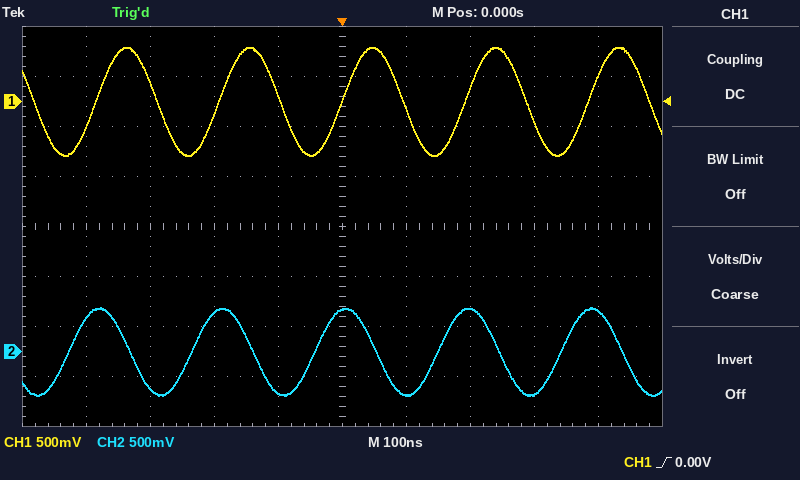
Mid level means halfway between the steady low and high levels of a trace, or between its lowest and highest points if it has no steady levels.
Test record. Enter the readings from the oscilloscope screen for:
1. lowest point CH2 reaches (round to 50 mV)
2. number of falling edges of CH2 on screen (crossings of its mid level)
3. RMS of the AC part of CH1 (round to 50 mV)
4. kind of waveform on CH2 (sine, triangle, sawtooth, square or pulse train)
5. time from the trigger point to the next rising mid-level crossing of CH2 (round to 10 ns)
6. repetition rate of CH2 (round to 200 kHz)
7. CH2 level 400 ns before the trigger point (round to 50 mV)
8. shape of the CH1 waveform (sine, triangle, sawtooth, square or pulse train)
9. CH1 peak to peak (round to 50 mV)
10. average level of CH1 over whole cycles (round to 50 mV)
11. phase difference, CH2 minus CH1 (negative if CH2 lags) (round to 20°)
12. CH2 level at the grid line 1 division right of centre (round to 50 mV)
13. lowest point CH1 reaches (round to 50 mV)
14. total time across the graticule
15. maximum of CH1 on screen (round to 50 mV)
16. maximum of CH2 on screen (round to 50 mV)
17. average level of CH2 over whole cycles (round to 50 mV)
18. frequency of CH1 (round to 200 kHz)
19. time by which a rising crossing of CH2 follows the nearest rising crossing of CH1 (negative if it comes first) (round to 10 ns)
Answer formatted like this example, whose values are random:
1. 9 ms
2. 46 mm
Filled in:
1. -450 mV
2. 5
3. 400 mV
4. sine
5. 150 ns
6. 5.2 MHz
7. 350 mV
8. sine
9. 1.10 V
10. 0 mV
11. +80°
12. -450 mV
13. -550 mV
14. 1 µs
15. 550 mV
16. 450 mV
17. 0 mV
18. 5.2 MHz
19. -40 ns
